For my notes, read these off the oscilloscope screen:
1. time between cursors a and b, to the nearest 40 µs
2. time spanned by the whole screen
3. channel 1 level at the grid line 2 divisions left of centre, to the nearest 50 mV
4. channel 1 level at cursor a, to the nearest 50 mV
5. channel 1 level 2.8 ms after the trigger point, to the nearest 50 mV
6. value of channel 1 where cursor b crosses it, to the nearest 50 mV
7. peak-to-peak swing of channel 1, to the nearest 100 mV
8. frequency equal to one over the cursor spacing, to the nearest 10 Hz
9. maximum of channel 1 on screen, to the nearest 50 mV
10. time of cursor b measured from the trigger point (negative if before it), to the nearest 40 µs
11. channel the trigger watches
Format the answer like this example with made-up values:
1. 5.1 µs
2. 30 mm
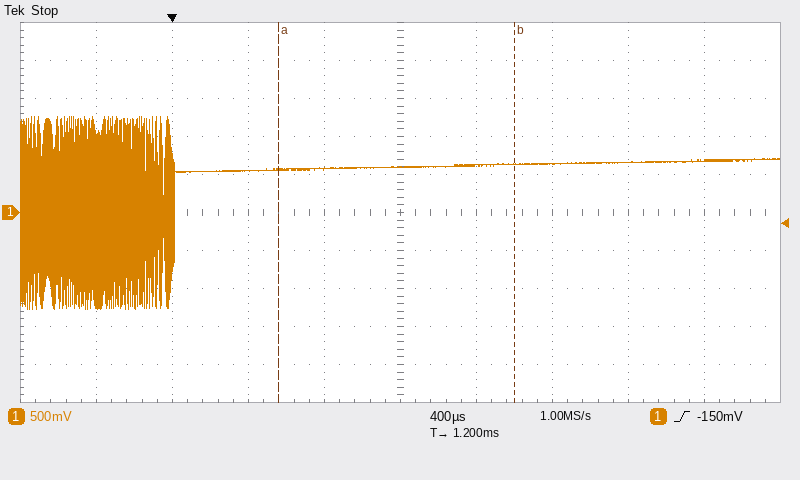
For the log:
1. 1.24 ms
2. 4 ms
3. 550 mV
4. 550 mV
5. 700 mV
6. 650 mV
7. 2.50 V
8. 810 Hz
9. 1.25 V
10. +1.80 ms
11. channel 1
